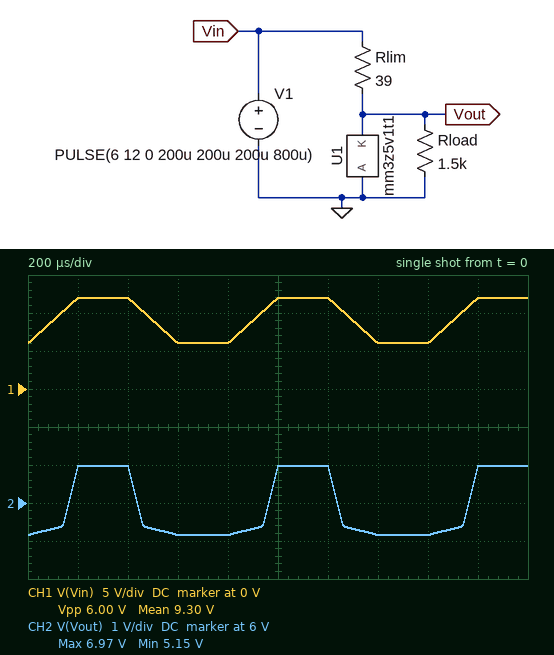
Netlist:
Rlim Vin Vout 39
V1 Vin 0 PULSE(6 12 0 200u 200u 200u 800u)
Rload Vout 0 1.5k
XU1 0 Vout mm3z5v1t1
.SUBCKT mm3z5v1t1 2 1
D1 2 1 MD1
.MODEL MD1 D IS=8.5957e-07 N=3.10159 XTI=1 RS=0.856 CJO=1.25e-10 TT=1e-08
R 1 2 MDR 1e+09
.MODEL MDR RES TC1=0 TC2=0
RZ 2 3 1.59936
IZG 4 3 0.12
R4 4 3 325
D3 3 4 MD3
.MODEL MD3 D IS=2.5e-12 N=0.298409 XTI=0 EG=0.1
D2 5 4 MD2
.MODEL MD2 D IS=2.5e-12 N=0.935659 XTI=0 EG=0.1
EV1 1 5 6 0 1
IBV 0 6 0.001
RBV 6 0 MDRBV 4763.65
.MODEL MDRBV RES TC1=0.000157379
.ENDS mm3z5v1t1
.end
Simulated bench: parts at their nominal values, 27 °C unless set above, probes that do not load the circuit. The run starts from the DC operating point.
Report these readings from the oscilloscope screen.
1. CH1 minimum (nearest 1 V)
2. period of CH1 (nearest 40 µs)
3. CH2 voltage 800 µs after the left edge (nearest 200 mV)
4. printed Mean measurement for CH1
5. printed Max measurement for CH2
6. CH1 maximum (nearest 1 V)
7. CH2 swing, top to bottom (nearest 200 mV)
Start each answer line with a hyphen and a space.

- 6 V
- 800 µs
- 5.2 V
- 9.30 V
- 6.97 V
- 12 V
- 1.8 V
